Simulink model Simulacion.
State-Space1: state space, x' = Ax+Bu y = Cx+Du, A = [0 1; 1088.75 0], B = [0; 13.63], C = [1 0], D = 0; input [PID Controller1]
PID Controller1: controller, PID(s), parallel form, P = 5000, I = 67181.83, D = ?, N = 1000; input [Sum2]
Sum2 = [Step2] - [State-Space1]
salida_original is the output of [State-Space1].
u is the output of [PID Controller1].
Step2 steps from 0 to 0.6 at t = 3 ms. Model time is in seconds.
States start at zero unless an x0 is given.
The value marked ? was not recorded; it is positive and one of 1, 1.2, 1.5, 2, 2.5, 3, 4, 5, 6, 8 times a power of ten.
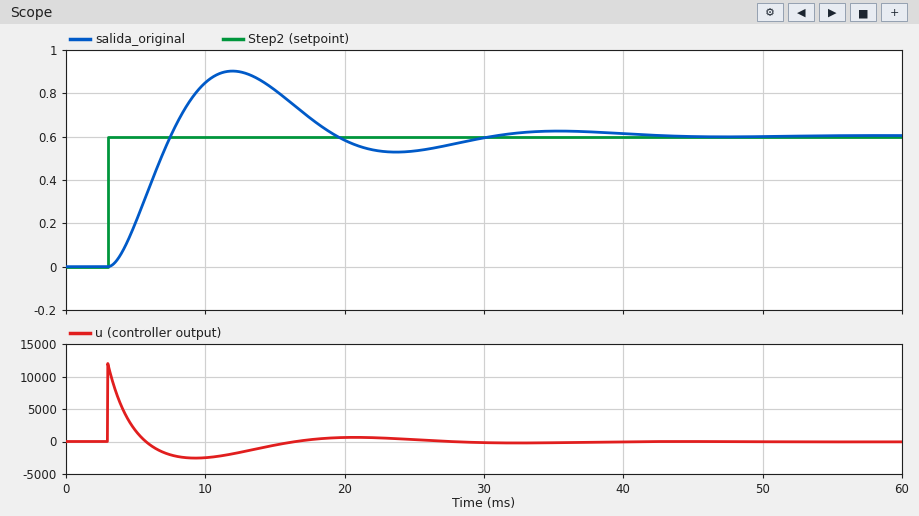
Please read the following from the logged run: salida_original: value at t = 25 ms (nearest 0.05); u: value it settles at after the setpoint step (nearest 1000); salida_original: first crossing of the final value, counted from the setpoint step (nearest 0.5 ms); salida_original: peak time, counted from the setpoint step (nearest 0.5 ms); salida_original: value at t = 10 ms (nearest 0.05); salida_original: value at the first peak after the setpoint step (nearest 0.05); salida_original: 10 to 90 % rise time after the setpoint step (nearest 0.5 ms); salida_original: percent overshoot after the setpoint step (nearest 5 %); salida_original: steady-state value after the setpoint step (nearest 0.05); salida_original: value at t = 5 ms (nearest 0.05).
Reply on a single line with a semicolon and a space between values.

0.55; 0; 4.5 ms; 9.0 ms; 0.85; 0.90; 3.0 ms; 50 %; 0.60; 0.20
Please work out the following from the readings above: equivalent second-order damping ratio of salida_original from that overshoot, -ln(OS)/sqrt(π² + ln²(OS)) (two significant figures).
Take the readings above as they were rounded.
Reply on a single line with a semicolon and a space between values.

0.22
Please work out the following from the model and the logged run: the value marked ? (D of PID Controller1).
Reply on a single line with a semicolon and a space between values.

15
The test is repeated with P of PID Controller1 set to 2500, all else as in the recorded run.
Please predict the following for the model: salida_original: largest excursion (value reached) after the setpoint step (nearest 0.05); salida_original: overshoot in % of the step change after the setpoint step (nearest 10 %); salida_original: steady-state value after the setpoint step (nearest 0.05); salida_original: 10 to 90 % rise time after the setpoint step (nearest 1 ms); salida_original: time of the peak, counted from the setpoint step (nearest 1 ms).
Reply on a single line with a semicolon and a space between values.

0.85; 40 %; 0.60; 4 ms; 12 ms
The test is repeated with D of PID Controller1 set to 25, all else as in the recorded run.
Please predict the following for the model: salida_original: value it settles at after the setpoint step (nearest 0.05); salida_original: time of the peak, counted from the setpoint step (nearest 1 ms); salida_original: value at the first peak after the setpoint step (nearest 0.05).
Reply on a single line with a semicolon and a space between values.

0.60; 7 ms; 0.80
